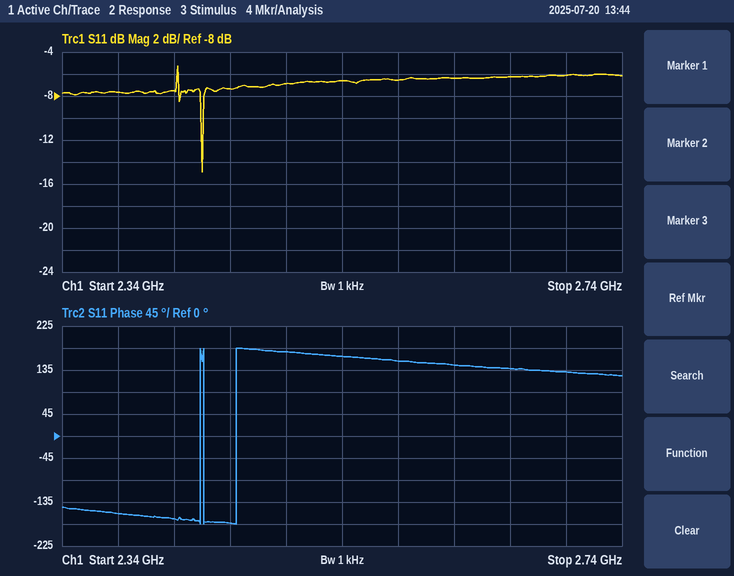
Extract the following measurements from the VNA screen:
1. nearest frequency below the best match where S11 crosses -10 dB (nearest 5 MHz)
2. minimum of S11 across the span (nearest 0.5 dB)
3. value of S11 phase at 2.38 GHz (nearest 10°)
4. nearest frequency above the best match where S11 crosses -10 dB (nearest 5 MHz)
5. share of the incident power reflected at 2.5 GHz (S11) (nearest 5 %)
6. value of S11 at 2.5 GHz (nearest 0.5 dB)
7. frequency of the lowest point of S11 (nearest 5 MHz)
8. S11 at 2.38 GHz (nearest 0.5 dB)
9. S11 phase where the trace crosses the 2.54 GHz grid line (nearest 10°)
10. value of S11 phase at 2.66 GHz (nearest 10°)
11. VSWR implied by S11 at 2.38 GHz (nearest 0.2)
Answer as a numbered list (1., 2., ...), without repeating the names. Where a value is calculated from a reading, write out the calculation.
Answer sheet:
1. 2.440 GHz
2. -15.0 dB
3. -160°
4. 2.440 GHz
5. 10^(-7/10) ≈ 20 %
6. -7.0 dB
7. 2.440 GHz
8. -7.5 dB
9. 160°
10. 140°
11. |Γ| = 10^(-7.5/20) = 0.4217; VSWR = (1 + 0.4217)/(1 − 0.4217) ≈ 2.46, so 2.4 to the nearest 0.2
